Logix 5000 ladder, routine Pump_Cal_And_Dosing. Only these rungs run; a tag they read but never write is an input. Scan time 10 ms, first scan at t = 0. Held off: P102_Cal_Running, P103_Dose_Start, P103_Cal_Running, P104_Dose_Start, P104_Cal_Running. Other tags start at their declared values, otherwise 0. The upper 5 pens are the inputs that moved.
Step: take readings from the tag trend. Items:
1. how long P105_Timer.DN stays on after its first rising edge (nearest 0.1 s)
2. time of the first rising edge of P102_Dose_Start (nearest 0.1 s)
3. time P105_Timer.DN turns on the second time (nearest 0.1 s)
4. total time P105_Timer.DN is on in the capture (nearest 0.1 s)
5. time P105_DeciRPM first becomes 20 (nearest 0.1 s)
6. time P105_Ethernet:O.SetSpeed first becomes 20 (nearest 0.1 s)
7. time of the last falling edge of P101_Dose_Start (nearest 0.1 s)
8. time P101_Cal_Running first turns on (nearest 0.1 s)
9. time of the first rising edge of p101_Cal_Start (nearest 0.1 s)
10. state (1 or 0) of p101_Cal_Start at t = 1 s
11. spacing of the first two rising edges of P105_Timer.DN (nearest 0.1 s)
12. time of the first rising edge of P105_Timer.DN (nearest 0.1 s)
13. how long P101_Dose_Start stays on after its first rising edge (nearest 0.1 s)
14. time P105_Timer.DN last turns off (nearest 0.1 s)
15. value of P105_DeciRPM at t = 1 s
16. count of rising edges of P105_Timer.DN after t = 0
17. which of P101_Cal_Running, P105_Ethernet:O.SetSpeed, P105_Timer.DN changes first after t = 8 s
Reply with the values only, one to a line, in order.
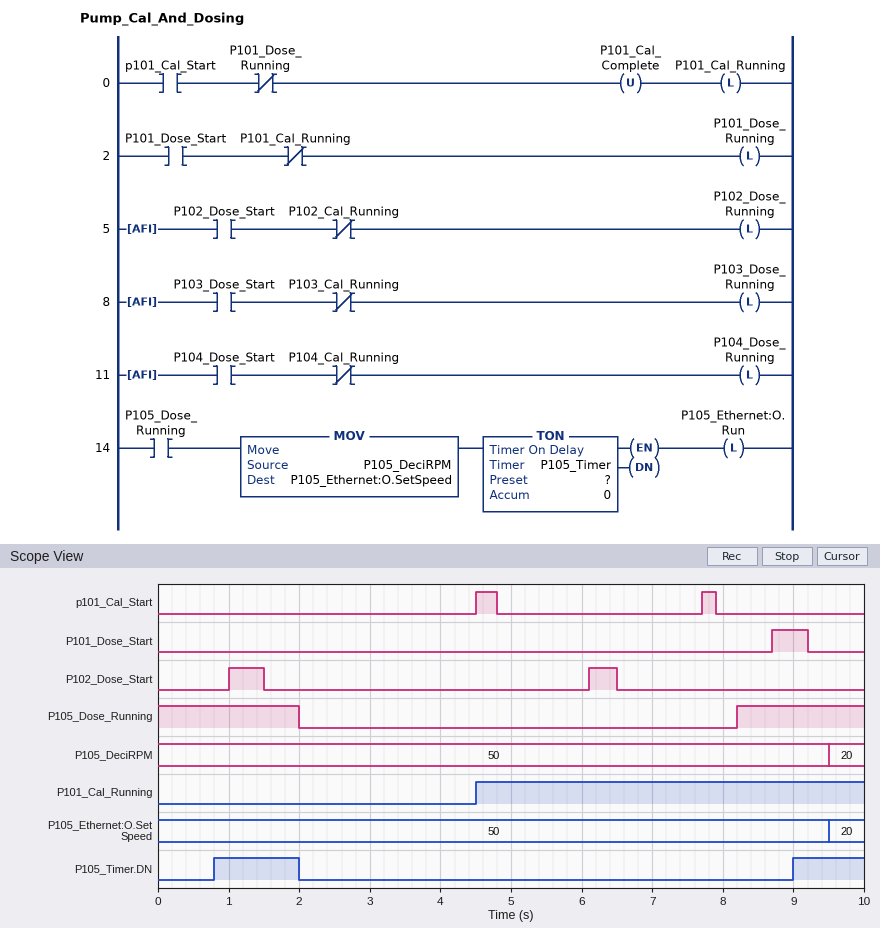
1.2 s
1.0 s
9.0 s
2.2 s
9.5 s
9.5 s
9.2 s
4.5 s
4.5 s
0
8.2 s
0.8 s
0.5 s
2.0 s
50
2
P105_Timer.DN
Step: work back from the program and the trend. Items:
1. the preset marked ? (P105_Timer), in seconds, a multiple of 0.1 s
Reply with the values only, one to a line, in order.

0.8 s
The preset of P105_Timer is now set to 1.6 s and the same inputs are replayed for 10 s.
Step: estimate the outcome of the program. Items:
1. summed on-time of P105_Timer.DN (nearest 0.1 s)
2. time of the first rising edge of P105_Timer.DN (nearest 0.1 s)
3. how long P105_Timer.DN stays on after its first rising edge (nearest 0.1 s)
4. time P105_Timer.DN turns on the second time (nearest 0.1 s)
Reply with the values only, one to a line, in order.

0.6 s
1.6 s
0.4 s
9.8 s
